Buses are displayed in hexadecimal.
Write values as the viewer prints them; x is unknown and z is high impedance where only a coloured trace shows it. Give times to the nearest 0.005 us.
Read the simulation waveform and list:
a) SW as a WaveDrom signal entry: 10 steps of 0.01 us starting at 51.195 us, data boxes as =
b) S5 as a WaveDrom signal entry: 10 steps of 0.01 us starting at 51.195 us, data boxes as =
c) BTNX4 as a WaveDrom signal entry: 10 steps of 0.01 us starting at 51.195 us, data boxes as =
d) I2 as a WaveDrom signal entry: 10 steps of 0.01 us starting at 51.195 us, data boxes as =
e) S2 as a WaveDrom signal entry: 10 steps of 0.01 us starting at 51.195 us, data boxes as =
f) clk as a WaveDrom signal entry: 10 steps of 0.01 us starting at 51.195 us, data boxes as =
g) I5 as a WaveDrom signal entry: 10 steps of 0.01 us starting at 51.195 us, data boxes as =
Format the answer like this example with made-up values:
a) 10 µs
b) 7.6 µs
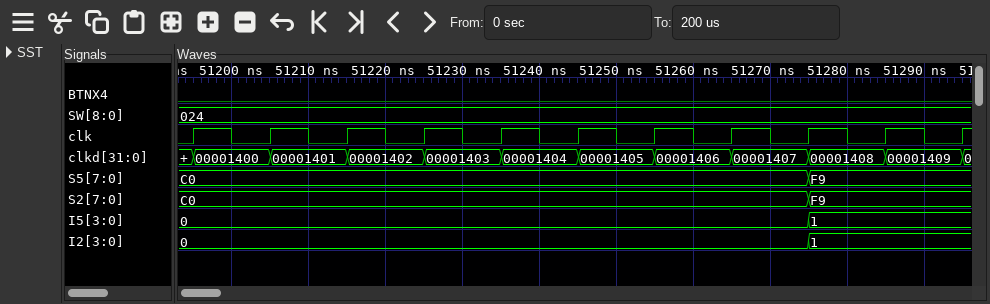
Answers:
a) {name: 'SW', wave: '=.........', data: '024'}
b) {name: 'S5', wave: '=.......=.', data: 'C0 F9'}
c) {name: 'BTNX4', wave: '0.........'}
d) {name: 'I2', wave: '=.......=.', data: '0 1'}
e) {name: 'S2', wave: '=.......=.', data: 'C0 F9'}
f) {name: 'clk', wave: 'p.........'}
g) {name: 'I5', wave: '=.......=.', data: '0 1'}
